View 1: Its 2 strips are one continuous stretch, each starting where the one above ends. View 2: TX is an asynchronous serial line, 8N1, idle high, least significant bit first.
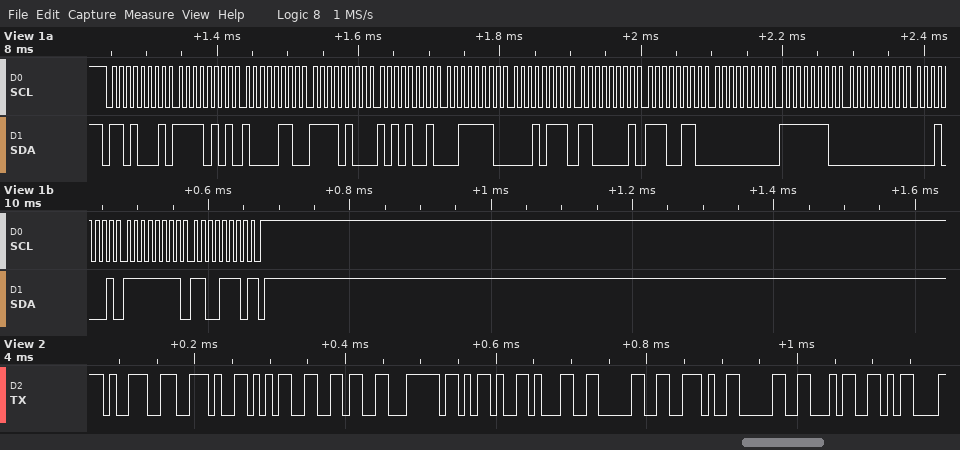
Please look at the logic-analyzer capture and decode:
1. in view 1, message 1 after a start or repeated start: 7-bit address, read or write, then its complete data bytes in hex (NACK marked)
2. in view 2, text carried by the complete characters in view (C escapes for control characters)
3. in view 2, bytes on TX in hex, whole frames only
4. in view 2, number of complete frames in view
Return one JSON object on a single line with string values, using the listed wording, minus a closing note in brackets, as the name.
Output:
{"in view 1, message 1 after a start or repeated start: 7-bit address, read or write, then its complete data bytes in hex": "0x68 read: F5 86 F4 A9 3E 17 C1 E6 00 FE 00 11 FF CE NACK", "in view 2, text carried by the complete characters in view": "\"9.56|-10.04\\r\"", "in view 2, bytes on TX in hex, whole frames only": "39 2E 35 36 7C 2D 31 30 2E 30 34 0D", "in view 2, number of complete frames in view": "12"}
